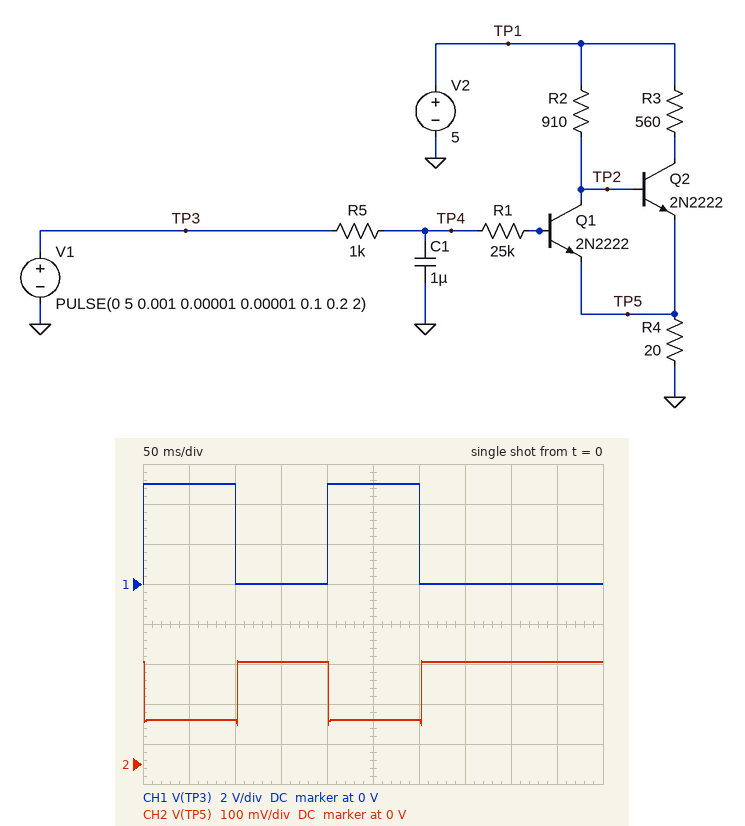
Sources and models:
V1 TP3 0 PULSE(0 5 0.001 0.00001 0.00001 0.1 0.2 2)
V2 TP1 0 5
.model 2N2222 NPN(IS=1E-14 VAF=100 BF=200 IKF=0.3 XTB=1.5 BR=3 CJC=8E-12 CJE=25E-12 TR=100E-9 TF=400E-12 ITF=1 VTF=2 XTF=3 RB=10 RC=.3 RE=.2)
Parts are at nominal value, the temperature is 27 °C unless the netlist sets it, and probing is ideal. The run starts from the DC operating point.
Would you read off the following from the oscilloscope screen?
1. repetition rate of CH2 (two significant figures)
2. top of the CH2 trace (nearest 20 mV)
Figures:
5.0 Hz
260 mV
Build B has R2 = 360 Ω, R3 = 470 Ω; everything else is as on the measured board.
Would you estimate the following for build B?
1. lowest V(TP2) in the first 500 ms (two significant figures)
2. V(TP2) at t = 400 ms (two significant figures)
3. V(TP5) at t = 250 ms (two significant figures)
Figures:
370 mV
1.3 V
260 mV
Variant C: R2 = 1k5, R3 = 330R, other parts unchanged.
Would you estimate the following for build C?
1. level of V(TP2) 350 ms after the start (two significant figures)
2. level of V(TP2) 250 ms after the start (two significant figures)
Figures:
1.1 V
130 mV
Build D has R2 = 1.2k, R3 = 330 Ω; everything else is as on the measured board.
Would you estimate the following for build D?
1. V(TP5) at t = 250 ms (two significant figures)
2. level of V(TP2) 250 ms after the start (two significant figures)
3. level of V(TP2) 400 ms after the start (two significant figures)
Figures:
84 mV
150 mV
1.1 V
